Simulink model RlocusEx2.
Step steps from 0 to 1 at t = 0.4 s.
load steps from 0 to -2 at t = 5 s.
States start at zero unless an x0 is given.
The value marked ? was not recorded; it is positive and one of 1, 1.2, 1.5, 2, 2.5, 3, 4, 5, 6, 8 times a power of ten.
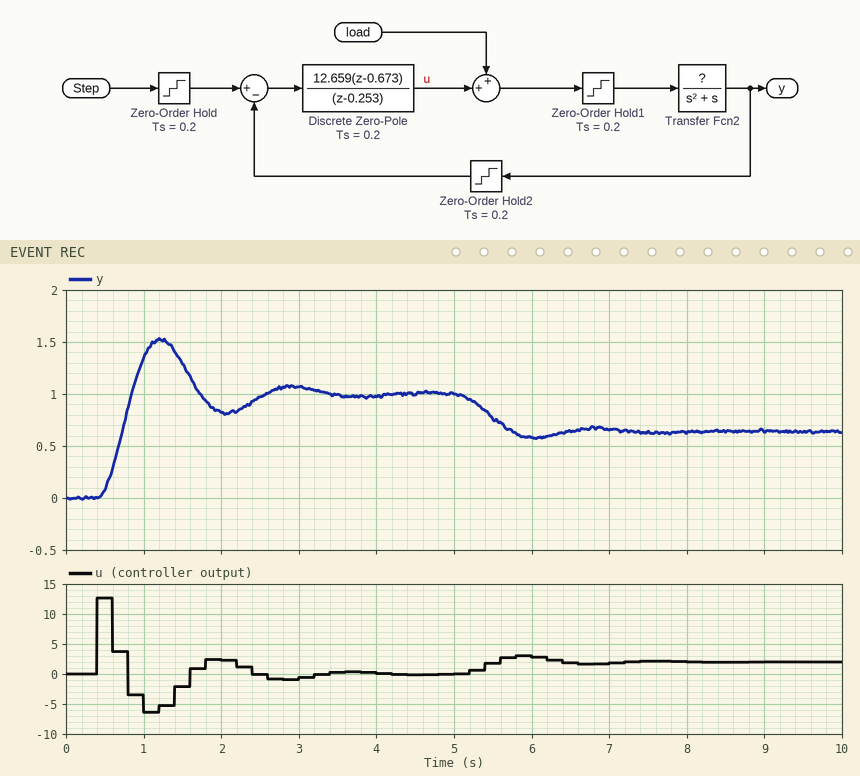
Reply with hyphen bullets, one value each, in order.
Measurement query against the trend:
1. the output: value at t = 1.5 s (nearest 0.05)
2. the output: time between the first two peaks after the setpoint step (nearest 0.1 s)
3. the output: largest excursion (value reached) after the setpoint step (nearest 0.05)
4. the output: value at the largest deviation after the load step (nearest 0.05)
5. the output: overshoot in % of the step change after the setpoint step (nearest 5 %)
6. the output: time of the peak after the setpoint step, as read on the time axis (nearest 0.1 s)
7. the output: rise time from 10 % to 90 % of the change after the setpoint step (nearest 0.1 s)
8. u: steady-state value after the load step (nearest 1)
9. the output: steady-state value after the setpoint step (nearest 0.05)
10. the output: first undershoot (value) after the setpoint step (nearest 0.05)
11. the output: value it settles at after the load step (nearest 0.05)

- 1.30
- 1.7 s
- 1.50
- 0.60
- 50 %
- 1.2 s
- 0.3 s
- 2
- 1.00
- 0.80
- 0.65
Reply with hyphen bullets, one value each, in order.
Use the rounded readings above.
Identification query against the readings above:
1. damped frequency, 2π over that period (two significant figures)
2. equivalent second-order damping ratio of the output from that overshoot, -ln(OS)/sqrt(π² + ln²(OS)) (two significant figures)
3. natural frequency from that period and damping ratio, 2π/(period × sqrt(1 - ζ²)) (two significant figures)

- 3.7 rad/s
- 0.22
- 3.8 rad/s
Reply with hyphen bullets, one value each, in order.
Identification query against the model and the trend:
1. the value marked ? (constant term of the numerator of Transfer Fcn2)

- 1.2
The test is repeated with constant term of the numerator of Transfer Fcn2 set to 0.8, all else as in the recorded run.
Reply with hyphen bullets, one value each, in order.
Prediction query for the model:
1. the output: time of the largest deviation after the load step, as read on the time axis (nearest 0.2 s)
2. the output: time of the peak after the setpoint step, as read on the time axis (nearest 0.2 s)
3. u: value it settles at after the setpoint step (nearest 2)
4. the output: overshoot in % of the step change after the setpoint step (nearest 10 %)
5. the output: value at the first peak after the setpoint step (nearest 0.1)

- 6.4 s
- 1.4 s
- 0
- 40 %
- 1.4
